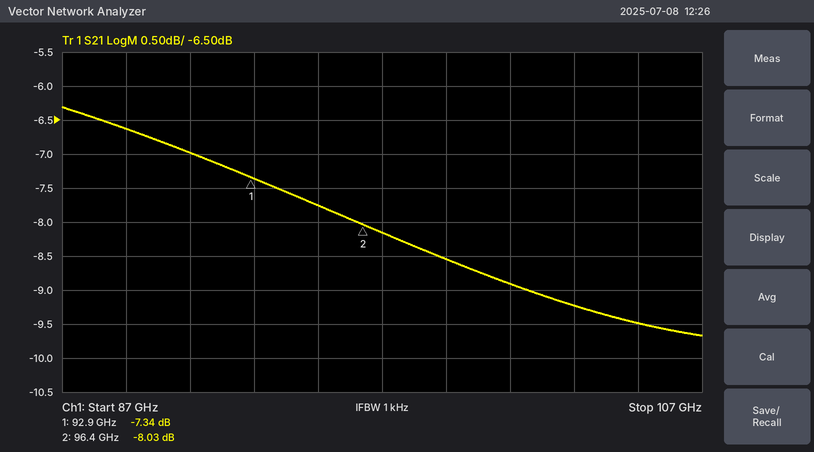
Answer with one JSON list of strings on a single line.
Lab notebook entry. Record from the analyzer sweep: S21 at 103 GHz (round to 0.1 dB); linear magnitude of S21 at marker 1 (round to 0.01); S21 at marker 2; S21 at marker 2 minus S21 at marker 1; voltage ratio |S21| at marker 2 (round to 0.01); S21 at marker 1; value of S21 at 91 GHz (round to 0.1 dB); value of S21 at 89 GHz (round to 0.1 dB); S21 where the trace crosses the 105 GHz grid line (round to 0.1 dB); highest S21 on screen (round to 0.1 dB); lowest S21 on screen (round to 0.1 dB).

["-9.2 dB", "0.43", "-8.03 dB", "-0.69 dB", "0.40", "-7.34 dB", "-7.0 dB", "-6.6 dB", "-9.5 dB", "-6.3 dB", "-9.7 dB"]
